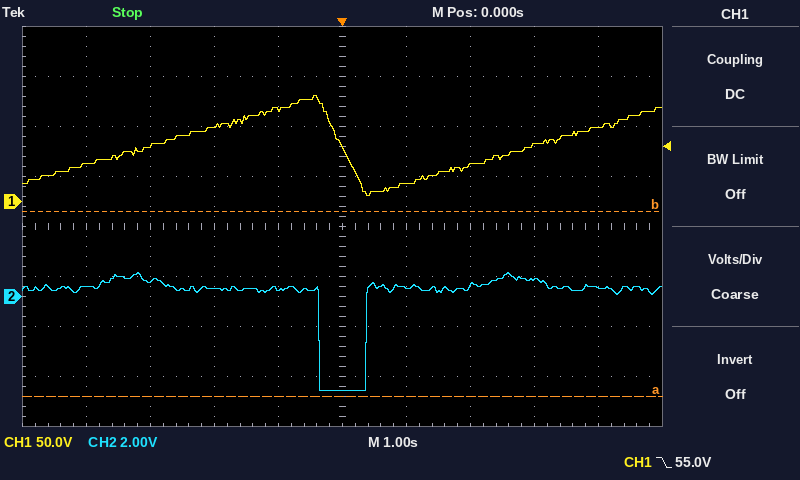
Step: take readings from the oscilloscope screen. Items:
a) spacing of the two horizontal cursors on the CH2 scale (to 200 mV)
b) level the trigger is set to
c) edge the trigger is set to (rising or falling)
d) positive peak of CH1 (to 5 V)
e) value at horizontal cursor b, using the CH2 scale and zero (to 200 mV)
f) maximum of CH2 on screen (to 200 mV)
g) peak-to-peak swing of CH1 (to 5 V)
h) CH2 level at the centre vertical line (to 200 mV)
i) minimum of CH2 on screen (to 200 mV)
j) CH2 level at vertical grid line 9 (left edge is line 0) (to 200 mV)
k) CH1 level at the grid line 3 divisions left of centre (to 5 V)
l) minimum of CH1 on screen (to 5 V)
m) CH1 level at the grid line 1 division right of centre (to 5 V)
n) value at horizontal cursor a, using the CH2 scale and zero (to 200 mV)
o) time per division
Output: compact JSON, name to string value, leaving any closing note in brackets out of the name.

{"spacing of the two horizontal cursors on the CH2 scale": "7.4 V", "level the trigger is set to": "55.0 V", "edge the trigger is set to": "falling", "positive peak of CH1": "105 V", "value at horizontal cursor b, using the CH2 scale and zero": "3.4 V", "maximum of CH2 on screen": "1.0 V", "peak-to-peak swing of CH1": "100 V", "CH2 level at the centre vertical line": "-3.8 V", "minimum of CH2 on screen": "-3.8 V", "CH2 level at vertical grid line 9 (left edge is line 0)": "400 mV", "CH1 level at the grid line 3 divisions left of centre": "55 V", "minimum of CH1 on screen": "5 V", "CH1 level at the grid line 1 division right of centre": "20 V", "value at horizontal cursor a, using the CH2 scale and zero": "-4.0 V", "time per division": "1 s"}
